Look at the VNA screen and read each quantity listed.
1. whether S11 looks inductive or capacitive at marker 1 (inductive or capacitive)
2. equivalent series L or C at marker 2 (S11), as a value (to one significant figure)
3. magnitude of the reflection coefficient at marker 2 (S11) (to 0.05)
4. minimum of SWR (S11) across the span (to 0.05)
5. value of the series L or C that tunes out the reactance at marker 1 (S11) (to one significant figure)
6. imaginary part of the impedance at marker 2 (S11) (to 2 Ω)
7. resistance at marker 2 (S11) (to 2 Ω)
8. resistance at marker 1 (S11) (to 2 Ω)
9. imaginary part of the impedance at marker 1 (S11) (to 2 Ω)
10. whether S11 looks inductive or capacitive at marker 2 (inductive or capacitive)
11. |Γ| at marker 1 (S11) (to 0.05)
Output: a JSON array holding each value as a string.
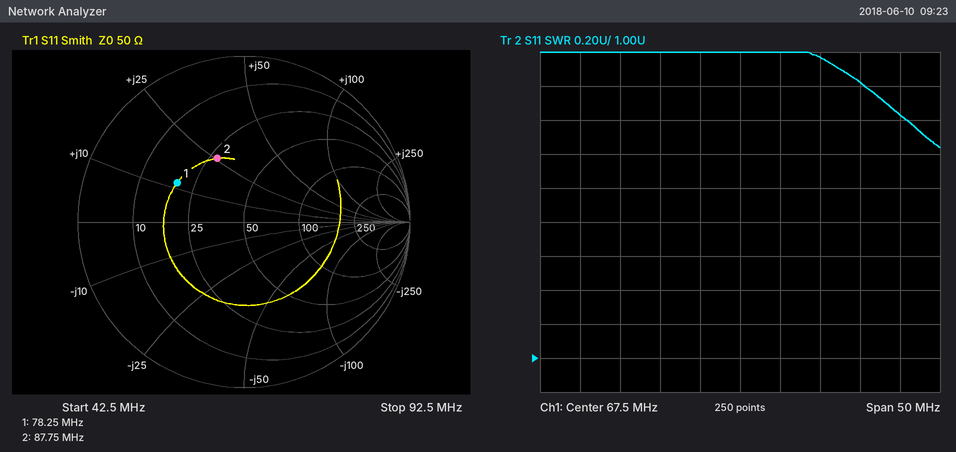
["inductive", "50 nH", "0.40", "2.25", "200 pF", "+26 Ω", "28 Ω", "20 Ω", "+12 Ω", "inductive", "0.45"]
